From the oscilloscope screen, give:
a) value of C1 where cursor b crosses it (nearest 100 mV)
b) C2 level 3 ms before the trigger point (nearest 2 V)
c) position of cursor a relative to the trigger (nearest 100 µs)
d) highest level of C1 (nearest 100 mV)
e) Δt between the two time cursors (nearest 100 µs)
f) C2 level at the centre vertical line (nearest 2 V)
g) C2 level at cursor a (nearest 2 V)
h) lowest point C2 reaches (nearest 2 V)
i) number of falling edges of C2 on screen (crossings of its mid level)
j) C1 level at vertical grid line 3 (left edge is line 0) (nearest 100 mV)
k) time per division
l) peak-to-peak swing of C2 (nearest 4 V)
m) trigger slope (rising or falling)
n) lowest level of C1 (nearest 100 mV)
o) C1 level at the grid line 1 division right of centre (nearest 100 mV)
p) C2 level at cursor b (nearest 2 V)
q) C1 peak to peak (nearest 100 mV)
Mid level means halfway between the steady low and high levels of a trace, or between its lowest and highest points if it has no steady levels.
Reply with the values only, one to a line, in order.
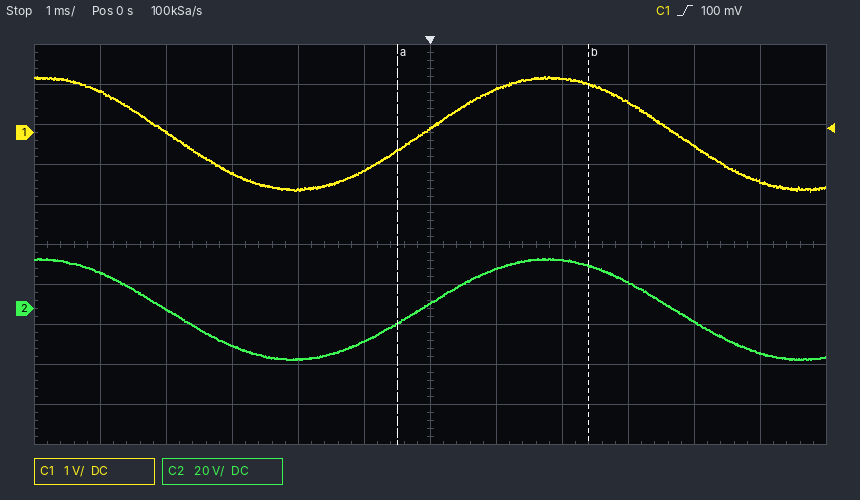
1.2 V
-18 V
-500 µs
1.4 V
2.9 ms
2 V
-8 V
-26 V
2
-1.0 V
1 ms
52 V
rising
-1.5 V
1.1 V
22 V
2.9 V
